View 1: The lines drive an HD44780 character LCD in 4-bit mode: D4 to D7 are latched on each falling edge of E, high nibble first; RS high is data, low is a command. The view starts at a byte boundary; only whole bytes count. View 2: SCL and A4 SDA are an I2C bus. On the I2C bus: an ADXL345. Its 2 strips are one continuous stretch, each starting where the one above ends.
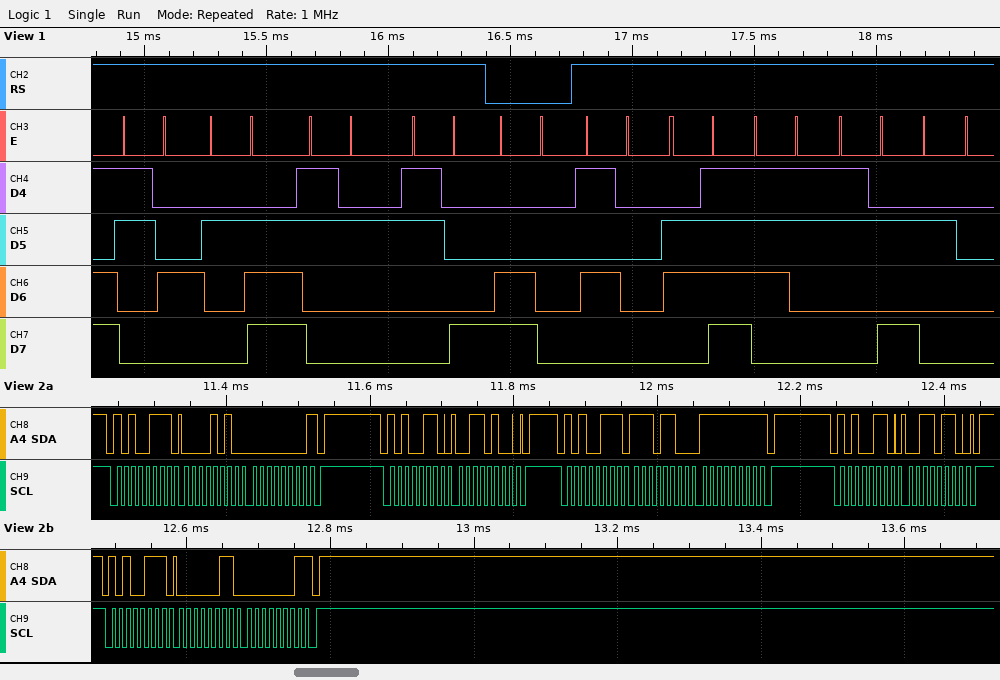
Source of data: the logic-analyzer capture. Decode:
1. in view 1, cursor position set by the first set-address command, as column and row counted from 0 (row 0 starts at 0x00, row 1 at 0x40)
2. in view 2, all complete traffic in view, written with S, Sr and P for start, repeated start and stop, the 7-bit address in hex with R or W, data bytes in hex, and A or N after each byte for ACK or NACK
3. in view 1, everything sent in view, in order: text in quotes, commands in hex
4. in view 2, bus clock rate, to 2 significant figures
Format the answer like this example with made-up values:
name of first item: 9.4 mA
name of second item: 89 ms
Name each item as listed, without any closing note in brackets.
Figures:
in view 1, cursor position set by the first set-address command, as column and row counted from 0: column 0, row 1
in view 2, all complete traffic in view, written with S, Sr and P for start, repeated start and stop, the 7-bit address in hex with R or W, data bytes in hex, and A or N after each byte for ACK or NACK: S 53R A 0A A 00 N P S 53W A 34 A P S 53R A EC A FF N P S 53W A 36 A P S 53R A 03 A 01 N P
in view 1, everything sent in view, in order: text in quotes, commands in hex: "4.28" 0xC0 "Pos: "
in view 2, bus clock rate, to 2 significant figures: 100 kHz
